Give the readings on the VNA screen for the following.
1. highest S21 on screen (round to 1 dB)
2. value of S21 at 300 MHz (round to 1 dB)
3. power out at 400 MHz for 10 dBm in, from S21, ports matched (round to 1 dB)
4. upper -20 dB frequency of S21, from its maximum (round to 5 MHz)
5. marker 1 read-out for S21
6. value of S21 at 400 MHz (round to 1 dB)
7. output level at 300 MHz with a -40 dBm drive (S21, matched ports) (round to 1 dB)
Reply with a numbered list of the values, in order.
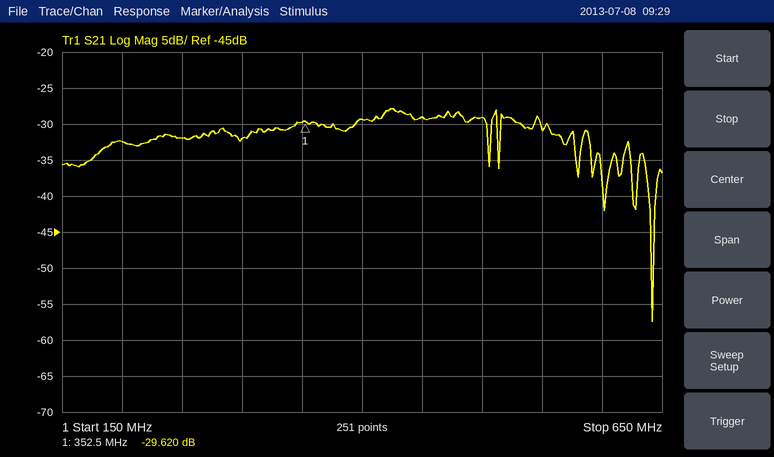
1. -28 dB
2. -32 dB
3. -19 dBm
4. 640 MHz
5. -29.620 dB
6. -29 dB
7. -72 dBm
